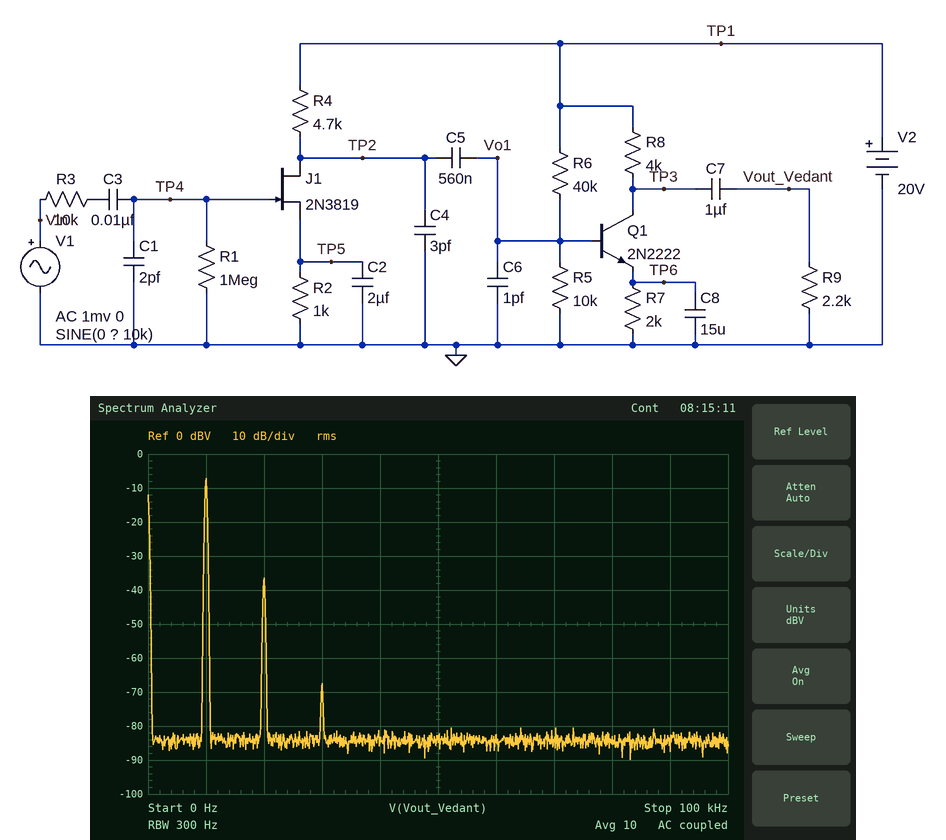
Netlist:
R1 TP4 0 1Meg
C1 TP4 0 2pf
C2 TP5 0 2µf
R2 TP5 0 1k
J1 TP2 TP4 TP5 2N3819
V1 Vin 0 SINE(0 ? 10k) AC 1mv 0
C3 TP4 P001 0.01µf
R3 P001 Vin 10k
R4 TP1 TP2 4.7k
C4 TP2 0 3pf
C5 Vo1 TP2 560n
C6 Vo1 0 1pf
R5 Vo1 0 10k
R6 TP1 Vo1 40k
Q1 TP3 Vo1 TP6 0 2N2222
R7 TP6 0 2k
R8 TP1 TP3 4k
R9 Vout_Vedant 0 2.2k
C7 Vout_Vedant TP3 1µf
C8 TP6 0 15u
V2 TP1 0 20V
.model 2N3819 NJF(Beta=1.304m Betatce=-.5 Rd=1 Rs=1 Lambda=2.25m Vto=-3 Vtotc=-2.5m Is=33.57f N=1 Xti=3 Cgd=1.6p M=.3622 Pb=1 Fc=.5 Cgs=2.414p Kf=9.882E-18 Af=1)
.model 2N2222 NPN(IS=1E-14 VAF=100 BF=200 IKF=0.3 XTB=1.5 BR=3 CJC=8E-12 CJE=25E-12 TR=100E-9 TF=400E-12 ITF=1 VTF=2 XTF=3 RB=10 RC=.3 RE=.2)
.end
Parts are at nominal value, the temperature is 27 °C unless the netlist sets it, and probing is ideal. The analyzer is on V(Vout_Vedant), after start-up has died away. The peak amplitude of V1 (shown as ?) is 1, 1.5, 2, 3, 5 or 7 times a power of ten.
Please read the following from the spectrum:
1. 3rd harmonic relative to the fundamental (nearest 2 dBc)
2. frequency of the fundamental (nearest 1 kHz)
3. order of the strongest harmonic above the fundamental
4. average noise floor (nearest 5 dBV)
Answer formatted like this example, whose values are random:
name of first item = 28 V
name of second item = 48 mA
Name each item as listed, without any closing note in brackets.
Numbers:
3rd harmonic relative to the fundamental = -60 dBc
frequency of the fundamental = 10 kHz
order of the strongest harmonic above the fundamental = 2
average noise floor = -85 dBV
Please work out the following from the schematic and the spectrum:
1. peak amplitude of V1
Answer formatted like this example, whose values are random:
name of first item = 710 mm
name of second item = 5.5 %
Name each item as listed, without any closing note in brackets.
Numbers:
peak amplitude of V1 = 1.5 mV
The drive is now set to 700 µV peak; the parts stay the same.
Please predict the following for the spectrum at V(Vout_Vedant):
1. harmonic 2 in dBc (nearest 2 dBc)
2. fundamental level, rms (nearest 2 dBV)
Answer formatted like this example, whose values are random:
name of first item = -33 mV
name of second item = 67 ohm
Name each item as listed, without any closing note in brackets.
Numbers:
harmonic 2 in dBc = -36 dBc
fundamental level, rms = -14 dBV
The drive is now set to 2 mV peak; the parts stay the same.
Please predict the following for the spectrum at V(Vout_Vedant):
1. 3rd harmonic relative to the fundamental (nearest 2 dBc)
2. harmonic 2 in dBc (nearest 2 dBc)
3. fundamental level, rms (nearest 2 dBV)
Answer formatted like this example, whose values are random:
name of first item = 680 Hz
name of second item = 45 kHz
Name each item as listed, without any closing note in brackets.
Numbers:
3rd harmonic relative to the fundamental = -56 dBc
harmonic 2 in dBc = -26 dBc
fundamental level, rms = -4 dBV
